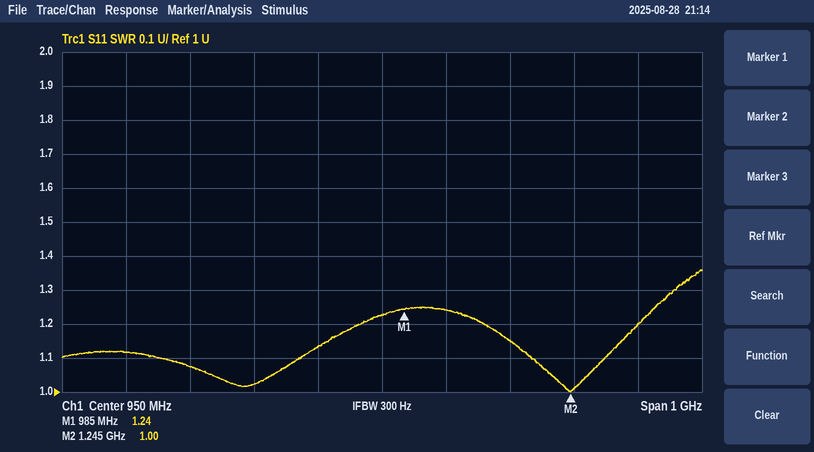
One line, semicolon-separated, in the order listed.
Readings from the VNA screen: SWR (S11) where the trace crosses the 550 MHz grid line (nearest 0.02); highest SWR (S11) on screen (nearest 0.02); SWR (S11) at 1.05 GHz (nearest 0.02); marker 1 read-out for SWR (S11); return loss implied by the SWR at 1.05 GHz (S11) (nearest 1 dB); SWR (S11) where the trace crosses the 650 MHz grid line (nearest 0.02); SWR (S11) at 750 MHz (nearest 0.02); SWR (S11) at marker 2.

1.12; 1.36; 1.24; 1.24; 19 dB; 1.08; 1.02; 1.00
